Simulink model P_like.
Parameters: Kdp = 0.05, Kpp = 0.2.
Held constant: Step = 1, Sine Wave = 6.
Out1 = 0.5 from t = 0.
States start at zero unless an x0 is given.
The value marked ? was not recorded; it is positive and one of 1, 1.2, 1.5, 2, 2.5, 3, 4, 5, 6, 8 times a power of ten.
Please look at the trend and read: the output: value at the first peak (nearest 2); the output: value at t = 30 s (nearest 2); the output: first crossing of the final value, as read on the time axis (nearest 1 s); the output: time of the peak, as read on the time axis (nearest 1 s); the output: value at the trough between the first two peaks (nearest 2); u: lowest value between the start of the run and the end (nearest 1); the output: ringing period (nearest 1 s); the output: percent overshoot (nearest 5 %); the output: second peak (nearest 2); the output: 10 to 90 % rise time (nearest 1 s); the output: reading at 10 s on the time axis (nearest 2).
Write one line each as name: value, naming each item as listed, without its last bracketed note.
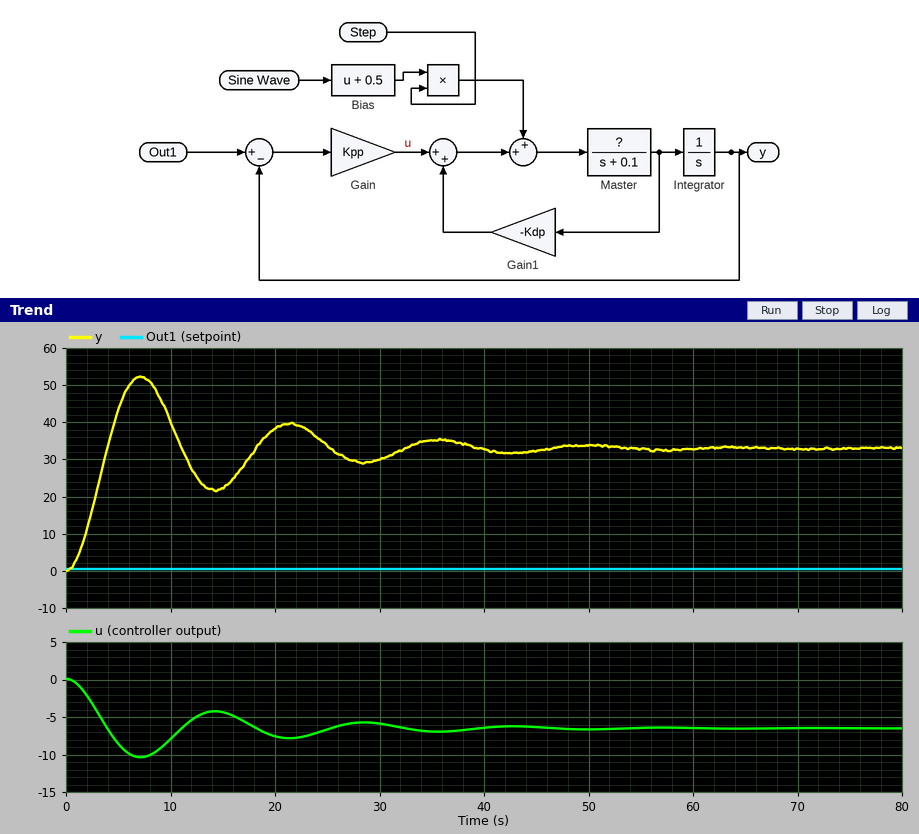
the output: value at the first peak: 52
the output: value at t = 30 s: 30
the output: first crossing of the final value, as read on the time axis: 4 s
the output: time of the peak, as read on the time axis: 7 s
the output: value at the trough between the first two peaks: 22
u: lowest value between the start of the run and the end: -10
the output: ringing period: 14 s
the output: percent overshoot: 60 %
the output: second peak: 40
the output: 10 to 90 % rise time: 3 s
the output: reading at 10 s on the time axis: 40
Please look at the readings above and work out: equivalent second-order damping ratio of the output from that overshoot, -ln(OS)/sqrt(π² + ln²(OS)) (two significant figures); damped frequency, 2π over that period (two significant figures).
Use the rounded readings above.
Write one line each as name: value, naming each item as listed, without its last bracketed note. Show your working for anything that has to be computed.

equivalent second-order damping ratio of the output from that overshoot, -ln(OS)/sqrt(π² + ln²(OS)): ln(0.6) = -0.511; 0.511 / sqrt(9.870 + 0.261) = 0.16
damped frequency, 2π over that period: 2π / 14 = 0.45 rad/s
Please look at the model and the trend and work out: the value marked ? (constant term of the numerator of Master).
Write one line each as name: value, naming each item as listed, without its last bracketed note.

the value marked ?: 1
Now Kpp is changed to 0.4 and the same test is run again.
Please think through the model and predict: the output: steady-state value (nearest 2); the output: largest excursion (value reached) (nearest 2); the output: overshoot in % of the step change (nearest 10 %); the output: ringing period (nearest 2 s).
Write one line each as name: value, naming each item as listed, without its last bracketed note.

the output: steady-state value: 16
the output: largest excursion (value reached): 28
the output: overshoot in % of the step change: 70 %
the output: ringing period: 10 s
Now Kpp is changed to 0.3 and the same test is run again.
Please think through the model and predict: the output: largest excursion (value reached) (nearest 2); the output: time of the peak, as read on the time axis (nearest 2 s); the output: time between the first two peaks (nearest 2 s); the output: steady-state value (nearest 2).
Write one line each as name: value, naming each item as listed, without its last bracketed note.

the output: largest excursion (value reached): 36
the output: time of the peak, as read on the time axis: 6 s
the output: time between the first two peaks: 12 s
the output: steady-state value: 22
